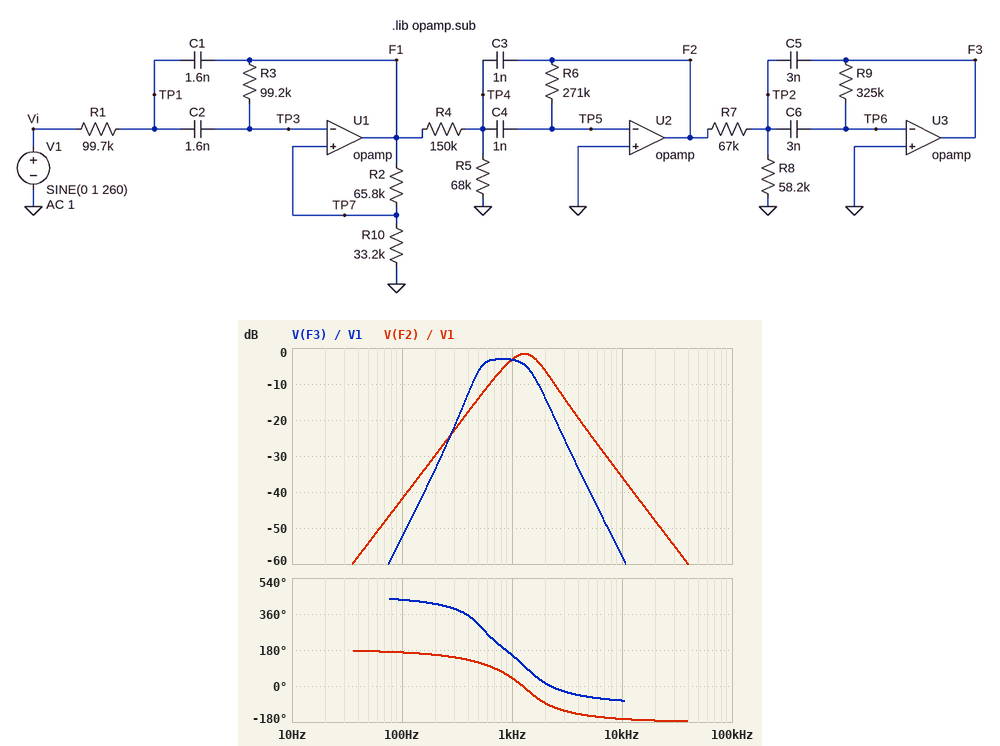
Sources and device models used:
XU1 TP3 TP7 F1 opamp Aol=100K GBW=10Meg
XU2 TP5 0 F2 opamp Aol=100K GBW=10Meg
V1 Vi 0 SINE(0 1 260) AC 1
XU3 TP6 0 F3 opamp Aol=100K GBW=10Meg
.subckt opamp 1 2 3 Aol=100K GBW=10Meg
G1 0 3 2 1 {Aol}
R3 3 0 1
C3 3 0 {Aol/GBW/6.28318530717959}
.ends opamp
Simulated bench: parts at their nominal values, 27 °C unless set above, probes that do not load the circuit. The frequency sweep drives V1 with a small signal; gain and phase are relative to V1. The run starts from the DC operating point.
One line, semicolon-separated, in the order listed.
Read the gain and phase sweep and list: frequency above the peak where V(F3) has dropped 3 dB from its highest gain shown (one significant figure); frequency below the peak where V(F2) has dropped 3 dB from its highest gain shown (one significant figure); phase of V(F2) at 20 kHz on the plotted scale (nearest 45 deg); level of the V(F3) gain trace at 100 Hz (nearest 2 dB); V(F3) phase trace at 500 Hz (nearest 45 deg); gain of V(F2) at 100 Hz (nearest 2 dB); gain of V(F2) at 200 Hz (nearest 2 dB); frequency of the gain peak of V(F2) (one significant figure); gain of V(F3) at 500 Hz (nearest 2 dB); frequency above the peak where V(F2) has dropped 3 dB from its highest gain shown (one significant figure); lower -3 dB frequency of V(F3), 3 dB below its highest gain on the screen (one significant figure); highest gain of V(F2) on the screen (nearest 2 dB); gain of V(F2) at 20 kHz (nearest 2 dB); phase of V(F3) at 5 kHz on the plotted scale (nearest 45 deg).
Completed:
1 kHz; 900 Hz; -180 deg; -52 dB; 315 deg; -42 dB; -30 dB; 1 kHz; -6 dB; 2 kHz; 500 Hz; -2 dB; -48 dB; -45 deg
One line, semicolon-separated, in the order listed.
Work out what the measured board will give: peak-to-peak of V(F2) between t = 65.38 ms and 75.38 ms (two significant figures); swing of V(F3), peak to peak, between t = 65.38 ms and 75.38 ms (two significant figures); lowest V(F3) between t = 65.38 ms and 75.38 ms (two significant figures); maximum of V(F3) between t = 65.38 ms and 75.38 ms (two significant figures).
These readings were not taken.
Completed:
110 mV; 99 mV; -49 mV; 49 mV
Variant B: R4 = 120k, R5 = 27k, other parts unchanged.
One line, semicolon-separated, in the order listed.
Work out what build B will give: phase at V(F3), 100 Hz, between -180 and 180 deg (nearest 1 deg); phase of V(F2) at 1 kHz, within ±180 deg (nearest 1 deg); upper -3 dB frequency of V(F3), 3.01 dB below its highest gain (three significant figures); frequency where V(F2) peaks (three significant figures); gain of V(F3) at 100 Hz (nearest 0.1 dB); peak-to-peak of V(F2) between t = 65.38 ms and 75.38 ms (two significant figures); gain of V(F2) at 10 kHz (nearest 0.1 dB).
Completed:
73 deg; 70 deg; 2.19 kHz; 1.92 kHz; -57.2 dB; 64 mV; -33.7 dB
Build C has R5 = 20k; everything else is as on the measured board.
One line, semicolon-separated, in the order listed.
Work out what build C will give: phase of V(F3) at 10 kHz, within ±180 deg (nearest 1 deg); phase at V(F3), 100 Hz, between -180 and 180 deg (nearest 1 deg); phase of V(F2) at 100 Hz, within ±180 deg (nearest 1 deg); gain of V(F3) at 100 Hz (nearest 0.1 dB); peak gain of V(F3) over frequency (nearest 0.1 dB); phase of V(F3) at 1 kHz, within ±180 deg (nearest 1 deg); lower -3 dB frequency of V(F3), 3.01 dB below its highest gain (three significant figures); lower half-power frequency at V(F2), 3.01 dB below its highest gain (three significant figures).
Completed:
-73 deg; 73 deg; 170 deg; -61.1 dB; -12.3 dB; -171 deg; 495 Hz; 1.55 kHz
